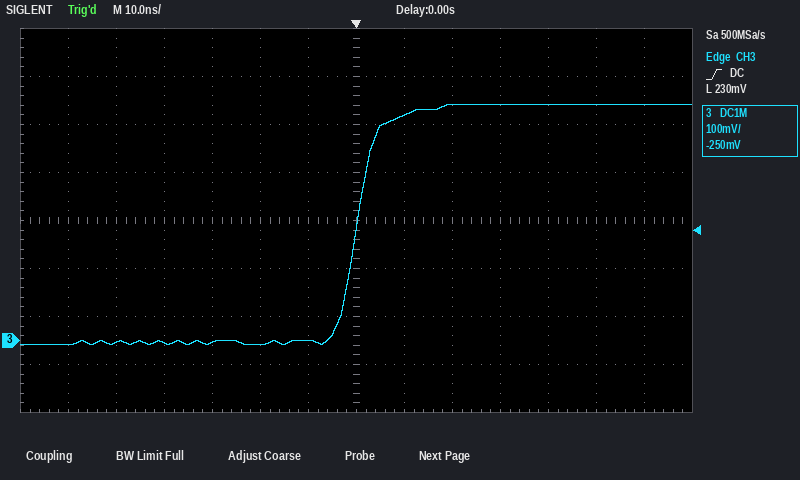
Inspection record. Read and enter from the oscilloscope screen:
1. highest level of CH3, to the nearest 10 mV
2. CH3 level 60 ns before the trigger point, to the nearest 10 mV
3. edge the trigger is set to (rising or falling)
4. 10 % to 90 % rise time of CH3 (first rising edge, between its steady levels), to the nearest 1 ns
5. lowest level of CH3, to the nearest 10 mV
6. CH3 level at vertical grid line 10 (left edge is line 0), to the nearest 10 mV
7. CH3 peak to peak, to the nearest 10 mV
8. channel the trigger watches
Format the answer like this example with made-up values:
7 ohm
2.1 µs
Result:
490 mV
-10 mV
rising
8 ns
-10 mV
490 mV
500 mV
CH3
